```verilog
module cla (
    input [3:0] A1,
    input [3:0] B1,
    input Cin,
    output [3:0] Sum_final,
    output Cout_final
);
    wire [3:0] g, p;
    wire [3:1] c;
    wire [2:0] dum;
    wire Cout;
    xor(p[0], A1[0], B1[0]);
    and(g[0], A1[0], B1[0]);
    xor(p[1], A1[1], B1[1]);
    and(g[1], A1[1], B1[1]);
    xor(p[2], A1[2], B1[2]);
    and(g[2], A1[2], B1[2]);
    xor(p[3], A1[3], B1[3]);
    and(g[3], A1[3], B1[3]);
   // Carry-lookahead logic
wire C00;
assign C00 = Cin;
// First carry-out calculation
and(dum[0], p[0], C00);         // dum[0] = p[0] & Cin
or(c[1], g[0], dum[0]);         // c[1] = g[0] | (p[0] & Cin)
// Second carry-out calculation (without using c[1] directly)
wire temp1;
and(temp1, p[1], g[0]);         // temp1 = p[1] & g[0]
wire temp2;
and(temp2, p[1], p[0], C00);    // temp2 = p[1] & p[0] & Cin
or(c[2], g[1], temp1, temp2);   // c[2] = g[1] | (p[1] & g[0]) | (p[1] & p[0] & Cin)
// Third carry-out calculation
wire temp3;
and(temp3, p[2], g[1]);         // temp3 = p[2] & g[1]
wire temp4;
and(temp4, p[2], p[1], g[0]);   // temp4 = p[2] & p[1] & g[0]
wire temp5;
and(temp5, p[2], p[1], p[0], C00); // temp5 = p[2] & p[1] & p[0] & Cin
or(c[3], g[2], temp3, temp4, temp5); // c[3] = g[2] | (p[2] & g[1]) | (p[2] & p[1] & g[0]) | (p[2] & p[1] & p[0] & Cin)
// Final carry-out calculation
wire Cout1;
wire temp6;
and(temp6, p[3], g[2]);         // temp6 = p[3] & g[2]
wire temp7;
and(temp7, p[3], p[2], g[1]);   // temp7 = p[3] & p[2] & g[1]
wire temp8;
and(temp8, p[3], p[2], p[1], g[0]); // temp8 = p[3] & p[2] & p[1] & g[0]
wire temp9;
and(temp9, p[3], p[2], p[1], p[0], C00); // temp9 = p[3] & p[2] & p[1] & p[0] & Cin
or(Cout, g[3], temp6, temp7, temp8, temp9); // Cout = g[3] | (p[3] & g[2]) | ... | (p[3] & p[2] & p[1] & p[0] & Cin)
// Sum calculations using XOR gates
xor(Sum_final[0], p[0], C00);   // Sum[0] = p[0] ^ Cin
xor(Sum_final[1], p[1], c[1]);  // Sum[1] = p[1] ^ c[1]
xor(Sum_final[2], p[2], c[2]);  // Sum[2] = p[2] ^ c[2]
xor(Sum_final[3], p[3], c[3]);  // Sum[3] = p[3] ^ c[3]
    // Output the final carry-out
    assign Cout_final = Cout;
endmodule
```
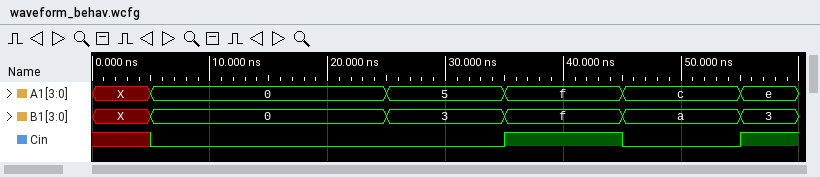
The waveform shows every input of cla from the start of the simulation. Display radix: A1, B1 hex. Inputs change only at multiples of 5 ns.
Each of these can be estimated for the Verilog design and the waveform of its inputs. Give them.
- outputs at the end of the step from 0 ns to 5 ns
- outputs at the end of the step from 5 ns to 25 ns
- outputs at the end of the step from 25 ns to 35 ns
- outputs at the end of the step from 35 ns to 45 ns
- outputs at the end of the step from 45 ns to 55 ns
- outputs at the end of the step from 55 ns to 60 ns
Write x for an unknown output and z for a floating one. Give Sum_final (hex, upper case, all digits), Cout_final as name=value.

Sum_final=x, Cout_final=x
Sum_final=0, Cout_final=0
Sum_final=8, Cout_final=0
Sum_final=F, Cout_final=1
Sum_final=6, Cout_final=1
Sum_final=2, Cout_final=1
